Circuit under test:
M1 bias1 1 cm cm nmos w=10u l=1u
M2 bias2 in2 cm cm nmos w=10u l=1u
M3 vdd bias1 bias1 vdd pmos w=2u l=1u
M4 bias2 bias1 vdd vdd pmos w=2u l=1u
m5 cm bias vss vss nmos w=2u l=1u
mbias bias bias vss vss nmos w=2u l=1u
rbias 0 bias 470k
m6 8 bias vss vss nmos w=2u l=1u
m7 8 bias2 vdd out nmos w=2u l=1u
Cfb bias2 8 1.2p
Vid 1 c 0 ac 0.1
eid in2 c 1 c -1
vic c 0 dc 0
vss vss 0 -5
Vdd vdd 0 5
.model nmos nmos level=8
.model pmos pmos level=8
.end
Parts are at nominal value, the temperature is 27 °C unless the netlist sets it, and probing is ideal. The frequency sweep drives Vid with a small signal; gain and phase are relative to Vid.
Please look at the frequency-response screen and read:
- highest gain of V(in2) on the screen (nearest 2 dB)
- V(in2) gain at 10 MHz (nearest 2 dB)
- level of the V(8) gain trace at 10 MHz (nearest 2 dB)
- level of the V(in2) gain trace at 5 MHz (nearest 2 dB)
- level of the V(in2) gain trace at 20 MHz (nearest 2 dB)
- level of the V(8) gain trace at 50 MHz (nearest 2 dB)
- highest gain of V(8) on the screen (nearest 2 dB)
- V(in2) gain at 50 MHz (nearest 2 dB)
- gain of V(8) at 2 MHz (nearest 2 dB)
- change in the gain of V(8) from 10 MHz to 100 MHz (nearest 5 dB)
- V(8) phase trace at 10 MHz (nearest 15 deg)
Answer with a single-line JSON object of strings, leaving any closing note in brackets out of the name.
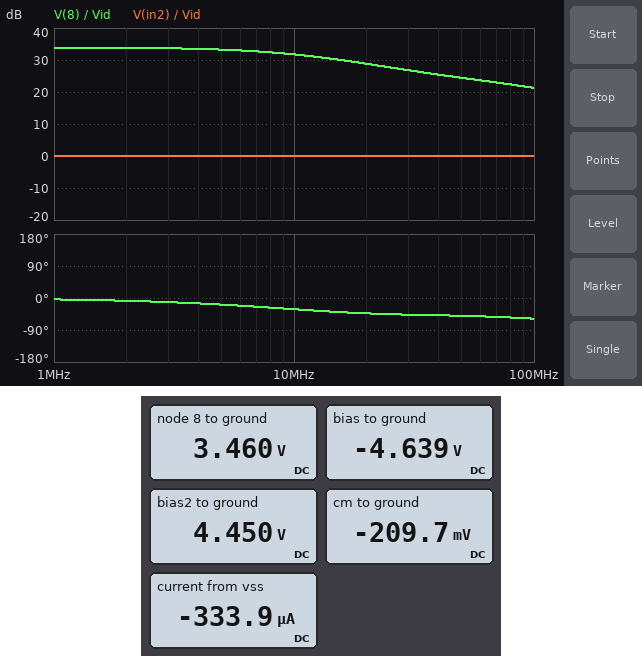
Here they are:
{"highest gain of V(in2) on the screen": "0 dB", "V(in2) gain at 10 MHz": "0 dB", "level of the V(8) gain trace at 10 MHz": "32 dB", "level of the V(in2) gain trace at 5 MHz": "0 dB", "level of the V(in2) gain trace at 20 MHz": "0 dB", "level of the V(8) gain trace at 50 MHz": "24 dB", "highest gain of V(8) on the screen": "34 dB", "V(in2) gain at 50 MHz": "0 dB", "gain of V(8) at 2 MHz": "34 dB", "change in the gain of V(8) from 10 MHz to 100 MHz": "-10 dB", "V(8) phase trace at 10 MHz": "-30 deg"}
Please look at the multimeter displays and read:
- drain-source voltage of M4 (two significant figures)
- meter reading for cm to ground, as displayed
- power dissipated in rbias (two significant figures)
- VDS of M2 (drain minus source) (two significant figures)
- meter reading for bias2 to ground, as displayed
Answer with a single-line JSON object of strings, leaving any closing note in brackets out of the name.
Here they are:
{"drain-source voltage of M4": "-550 mV", "meter reading for cm to ground, as displayed": "-209.7 mV", "power dissipated in rbias": "46 µW", "VDS of M2 (drain minus source)": "4.7 V", "meter reading for bias2 to ground, as displayed": "4.450 V"}
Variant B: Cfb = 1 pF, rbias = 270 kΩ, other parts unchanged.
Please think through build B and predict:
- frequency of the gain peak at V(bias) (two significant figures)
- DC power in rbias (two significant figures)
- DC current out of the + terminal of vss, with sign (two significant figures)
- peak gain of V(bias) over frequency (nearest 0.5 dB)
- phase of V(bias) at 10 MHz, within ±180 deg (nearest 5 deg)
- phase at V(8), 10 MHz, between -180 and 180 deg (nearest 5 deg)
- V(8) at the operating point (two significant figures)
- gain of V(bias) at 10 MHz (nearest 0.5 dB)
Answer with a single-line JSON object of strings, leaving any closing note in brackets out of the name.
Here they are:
{"frequency of the gain peak at V(bias)": "390 MHz", "DC power in rbias": "78 µW", "DC current out of the + terminal of vss, with sign": "-460 µA", "peak gain of V(bias) over frequency": "-20.0 dB", "phase of V(bias) at 10 MHz, within ±180 deg": "55 deg", "phase at V(8), 10 MHz, between -180 and 180 deg": "-35 deg", "V(8) at the operating point": "3.1 V", "gain of V(bias) at 10 MHz": "-32.5 dB"}
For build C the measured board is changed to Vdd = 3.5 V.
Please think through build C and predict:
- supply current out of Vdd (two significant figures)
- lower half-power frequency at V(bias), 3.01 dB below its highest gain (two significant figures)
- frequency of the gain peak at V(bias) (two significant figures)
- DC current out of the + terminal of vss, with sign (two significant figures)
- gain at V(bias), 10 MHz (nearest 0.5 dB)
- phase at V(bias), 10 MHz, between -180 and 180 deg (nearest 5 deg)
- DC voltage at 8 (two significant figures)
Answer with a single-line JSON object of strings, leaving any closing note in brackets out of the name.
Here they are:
{"supply current out of Vdd": "210 µA", "lower half-power frequency at V(bias), 3.01 dB below its highest gain": "100 MHz", "frequency of the gain peak at V(bias)": "300 MHz", "DC current out of the + terminal of vss, with sign": "-220 µA", "gain at V(bias), 10 MHz": "-30.0 dB", "phase at V(bias), 10 MHz, between -180 and 180 deg": "40 deg", "DC voltage at 8": "2.2 V"}
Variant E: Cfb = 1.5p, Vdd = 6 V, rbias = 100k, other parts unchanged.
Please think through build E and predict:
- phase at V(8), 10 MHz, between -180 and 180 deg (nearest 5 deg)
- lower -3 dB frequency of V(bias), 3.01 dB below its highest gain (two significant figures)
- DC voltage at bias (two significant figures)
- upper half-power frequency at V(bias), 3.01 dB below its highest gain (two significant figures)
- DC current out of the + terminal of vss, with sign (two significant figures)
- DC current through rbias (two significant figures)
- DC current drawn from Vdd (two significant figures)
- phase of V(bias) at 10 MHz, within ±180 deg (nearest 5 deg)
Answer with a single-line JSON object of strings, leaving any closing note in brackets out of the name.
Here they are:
{"phase at V(8), 10 MHz, between -180 and 180 deg": "-35 deg", "lower -3 dB frequency of V(bias), 3.01 dB below its highest gain": "270 MHz", "DC voltage at bias": "-4.5 V", "upper half-power frequency at V(bias), 3.01 dB below its highest gain": "3.2 GHz", "DC current out of the + terminal of vss, with sign": "-1.0 mA", "DC current through rbias": "45 µA", "DC current drawn from Vdd": "960 µA", "phase of V(bias) at 10 MHz, within ±180 deg": "55 deg"}
